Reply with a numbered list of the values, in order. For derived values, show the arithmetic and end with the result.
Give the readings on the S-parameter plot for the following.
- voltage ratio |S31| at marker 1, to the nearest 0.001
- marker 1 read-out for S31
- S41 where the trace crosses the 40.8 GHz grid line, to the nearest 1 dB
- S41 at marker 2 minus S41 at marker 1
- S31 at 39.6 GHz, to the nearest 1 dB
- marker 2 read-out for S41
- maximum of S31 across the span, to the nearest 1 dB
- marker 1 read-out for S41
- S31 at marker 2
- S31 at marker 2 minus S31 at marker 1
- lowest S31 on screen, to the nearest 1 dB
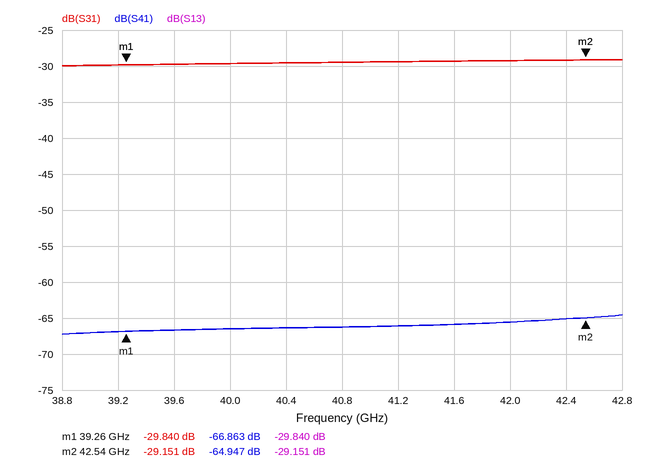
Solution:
1. 10^(-29.84/20) ≈ 0.032
2. -29.840 dB
3. -66 dB
4. -64.947 − (-66.863) = 1.916 dB
5. -30 dB
6. -64.947 dB
7. -29 dB
8. -66.863 dB
9. -29.151 dB
10. -29.151 − (-29.84) = 0.689 dB
11. -30 dB
